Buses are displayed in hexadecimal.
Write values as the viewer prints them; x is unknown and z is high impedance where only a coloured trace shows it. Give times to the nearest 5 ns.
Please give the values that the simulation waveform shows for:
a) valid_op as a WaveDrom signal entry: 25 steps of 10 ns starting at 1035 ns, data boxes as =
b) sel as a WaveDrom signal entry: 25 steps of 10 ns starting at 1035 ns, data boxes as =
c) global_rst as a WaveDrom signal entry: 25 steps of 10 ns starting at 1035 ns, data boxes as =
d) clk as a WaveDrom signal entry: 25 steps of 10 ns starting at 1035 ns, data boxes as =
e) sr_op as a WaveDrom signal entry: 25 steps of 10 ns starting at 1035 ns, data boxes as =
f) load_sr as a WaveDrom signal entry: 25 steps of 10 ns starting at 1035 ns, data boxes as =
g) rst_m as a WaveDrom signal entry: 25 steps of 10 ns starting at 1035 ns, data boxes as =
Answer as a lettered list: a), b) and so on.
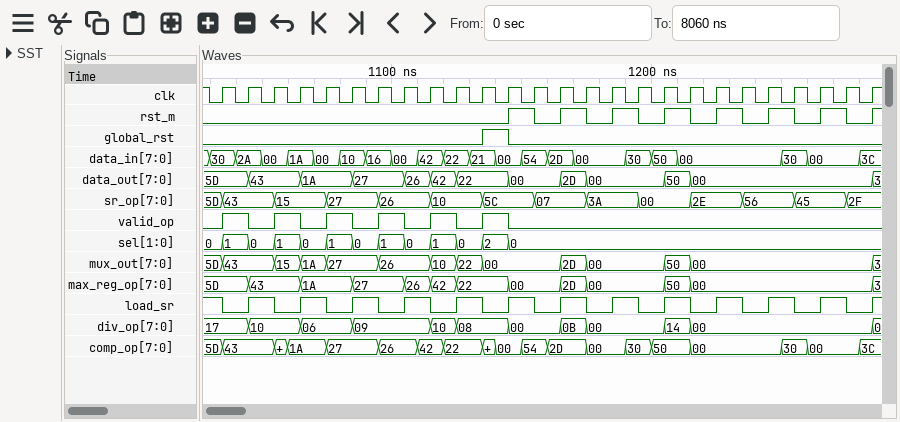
a) {name: 'valid_op', wave: '101010101010.............'}
b) {name: 'sel', wave: '============.............', data: '1 0 1 0 1 0 1 0 1 0 2 0'}
c) {name: 'global_rst', wave: '0.........10.............'}
d) {name: 'clk', wave: 'p........................'}
e) {name: 'sr_op', wave: '=.=.=.=.=.=.=.=.=.=.=.=.=', data: '43 15 27 26 10 5C 07 3A 00 2E 56 45 2F'}
f) {name: 'load_sr', wave: '0101010101010101010101010'}
g) {name: 'rst_m', wave: '0..........10101010101010'}
